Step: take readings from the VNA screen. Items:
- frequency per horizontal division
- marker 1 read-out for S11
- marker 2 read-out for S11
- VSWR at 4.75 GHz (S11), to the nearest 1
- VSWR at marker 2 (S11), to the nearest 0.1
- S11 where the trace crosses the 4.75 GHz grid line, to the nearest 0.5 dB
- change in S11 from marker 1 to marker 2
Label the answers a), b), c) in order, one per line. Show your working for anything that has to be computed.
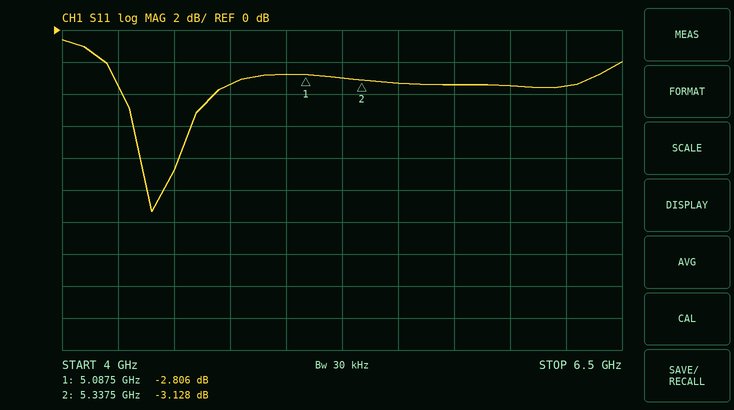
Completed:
a) 250 MHz
b) -2.806 dB
c) -3.128 dB
d) |Γ| = 10^(-3.5/20) = 0.6683; VSWR = (1 + 0.6683)/(1 − 0.6683) ≈ 5
e) (1 + 0.6976)/(1 − 0.6976) ≈ 5.6
f) -3.5 dB
g) -3.128 − (-2.806) = -0.322 dB
